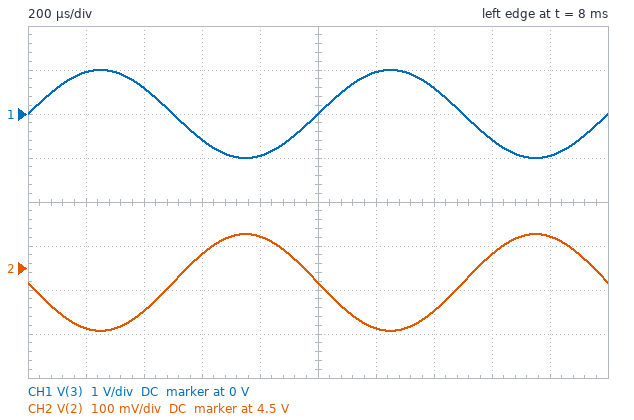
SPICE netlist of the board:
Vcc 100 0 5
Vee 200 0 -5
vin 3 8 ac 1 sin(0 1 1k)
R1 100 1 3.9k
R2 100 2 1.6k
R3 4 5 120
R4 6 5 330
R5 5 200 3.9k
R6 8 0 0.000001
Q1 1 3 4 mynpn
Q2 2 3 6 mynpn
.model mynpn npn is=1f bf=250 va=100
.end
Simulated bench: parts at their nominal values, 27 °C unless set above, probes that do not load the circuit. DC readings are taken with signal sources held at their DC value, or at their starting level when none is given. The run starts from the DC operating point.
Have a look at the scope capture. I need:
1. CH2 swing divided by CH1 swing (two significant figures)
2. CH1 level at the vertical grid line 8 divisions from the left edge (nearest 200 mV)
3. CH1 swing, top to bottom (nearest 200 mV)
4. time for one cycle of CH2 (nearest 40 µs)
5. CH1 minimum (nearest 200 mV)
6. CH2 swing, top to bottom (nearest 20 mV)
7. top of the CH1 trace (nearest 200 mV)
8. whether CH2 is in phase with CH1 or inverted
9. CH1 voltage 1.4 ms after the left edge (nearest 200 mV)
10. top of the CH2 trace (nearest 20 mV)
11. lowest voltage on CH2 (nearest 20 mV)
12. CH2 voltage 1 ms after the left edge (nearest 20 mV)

0.11
-600 mV
2.0 V
1.00 ms
-1.0 V
220 mV
1.0 V
inverted
600 mV
4.58 V
4.36 V
4.46 V
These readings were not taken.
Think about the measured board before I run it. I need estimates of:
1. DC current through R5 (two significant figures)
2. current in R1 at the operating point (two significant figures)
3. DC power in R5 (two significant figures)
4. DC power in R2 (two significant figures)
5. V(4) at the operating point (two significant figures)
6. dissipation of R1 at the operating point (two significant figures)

1.1 mA
740 µA
4.5 mW
180 µW
-710 mV
2.1 mW
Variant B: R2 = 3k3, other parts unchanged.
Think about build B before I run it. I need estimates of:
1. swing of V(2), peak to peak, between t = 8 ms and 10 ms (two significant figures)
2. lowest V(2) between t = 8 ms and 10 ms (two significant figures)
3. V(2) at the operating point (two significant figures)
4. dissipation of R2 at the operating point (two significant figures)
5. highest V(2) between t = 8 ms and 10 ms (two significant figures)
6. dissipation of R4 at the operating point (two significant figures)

450 mV
3.7 V
3.9 V
370 µW
4.1 V
37 µW
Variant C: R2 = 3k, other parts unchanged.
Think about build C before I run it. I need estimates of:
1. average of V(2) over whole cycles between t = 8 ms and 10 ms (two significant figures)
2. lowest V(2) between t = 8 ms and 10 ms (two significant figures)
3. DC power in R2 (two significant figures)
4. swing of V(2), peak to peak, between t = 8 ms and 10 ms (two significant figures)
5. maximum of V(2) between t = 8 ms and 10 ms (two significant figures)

4.0 V
3.8 V
330 µW
410 mV
4.2 V
